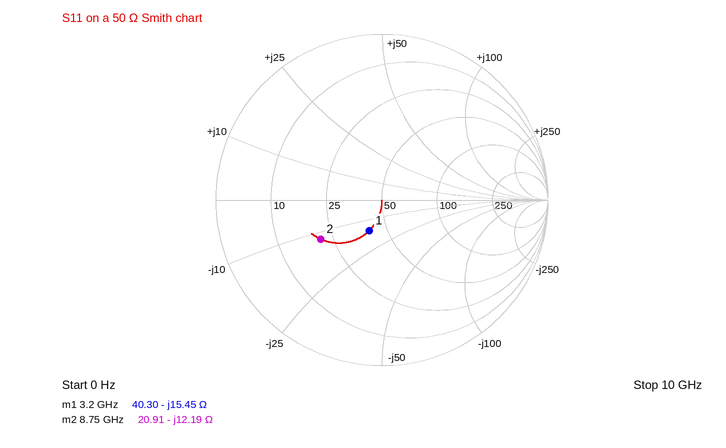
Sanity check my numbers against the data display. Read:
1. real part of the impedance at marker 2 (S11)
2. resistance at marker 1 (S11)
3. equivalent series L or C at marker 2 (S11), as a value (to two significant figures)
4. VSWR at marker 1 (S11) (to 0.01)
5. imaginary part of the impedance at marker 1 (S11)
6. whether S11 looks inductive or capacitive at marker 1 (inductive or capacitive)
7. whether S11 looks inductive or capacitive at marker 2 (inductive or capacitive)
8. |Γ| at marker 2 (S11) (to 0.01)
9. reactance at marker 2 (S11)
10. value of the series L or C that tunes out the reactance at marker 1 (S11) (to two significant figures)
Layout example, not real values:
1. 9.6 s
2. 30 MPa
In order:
1. 20.91 Ω
2. 40.30 Ω
3. 1.5 pF
4. 1.50
5. -15.45 Ω
6. capacitive
7. capacitive
8. 0.44
9. -12.19 Ω
10. 770 pH
